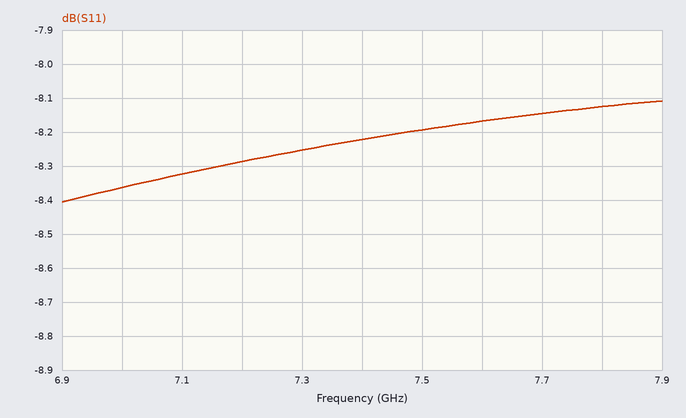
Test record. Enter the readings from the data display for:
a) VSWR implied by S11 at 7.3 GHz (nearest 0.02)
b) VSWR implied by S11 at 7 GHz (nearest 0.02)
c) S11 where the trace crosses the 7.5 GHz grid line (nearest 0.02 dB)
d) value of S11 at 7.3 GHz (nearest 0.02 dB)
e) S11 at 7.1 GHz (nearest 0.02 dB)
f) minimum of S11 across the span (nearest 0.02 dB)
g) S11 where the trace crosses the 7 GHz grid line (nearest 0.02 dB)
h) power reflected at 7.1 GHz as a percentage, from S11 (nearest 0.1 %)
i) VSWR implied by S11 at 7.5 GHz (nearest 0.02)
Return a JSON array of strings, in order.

["2.26", "2.24", "-8.20 dB", "-8.26 dB", "-8.32 dB", "-8.40 dB", "-8.36 dB", "14.7 %", "2.28"]
